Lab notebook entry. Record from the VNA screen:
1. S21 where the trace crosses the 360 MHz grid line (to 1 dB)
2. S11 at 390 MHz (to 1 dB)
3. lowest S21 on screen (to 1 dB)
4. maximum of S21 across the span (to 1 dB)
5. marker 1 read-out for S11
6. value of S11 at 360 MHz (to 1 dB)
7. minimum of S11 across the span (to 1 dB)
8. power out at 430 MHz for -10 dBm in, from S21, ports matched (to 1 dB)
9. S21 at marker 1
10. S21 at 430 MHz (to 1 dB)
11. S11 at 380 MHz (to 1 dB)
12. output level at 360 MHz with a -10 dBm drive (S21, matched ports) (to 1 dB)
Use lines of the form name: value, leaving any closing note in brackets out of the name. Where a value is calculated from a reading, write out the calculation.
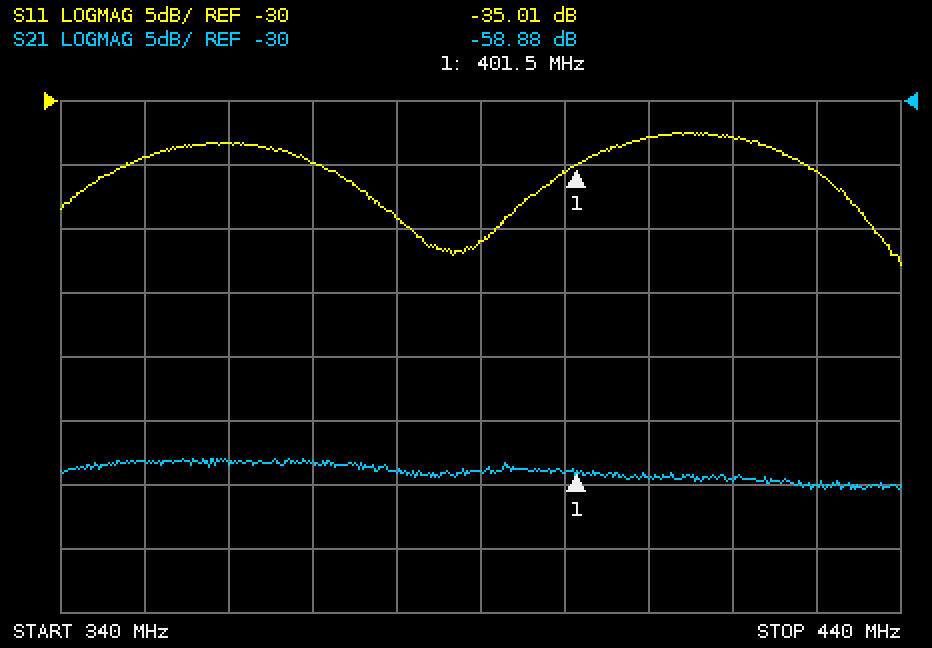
S21 where the trace crosses the 360 MHz grid line: -58 dB
S11 at 390 MHz: -41 dB
lowest S21 on screen: -60 dB
maximum of S21 across the span: -58 dB
marker 1 read-out for S11: -35.01 dB
value of S11 at 360 MHz: -33 dB
minimum of S11 across the span: -43 dB
power out at 430 MHz for -10 dBm in, from S21, ports matched: -10 dBm + (-60 dB) = -70 dBm
S21 at marker 1: -58.88 dB
S21 at 430 MHz: -60 dB
S11 at 380 MHz: -39 dB
output level at 360 MHz with a -10 dBm drive (S21, matched ports): -10 dBm + (-58 dB) = -68 dBm
